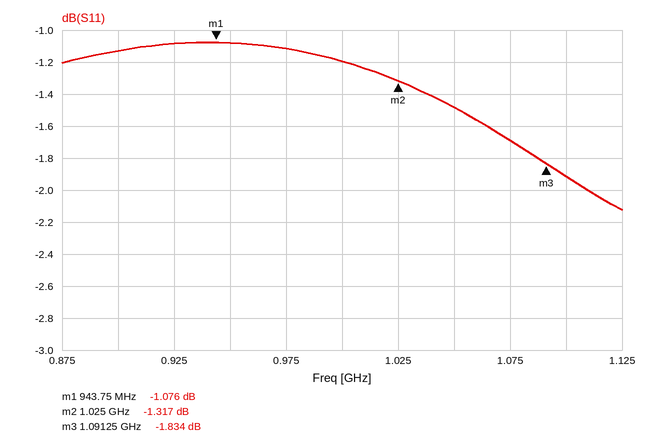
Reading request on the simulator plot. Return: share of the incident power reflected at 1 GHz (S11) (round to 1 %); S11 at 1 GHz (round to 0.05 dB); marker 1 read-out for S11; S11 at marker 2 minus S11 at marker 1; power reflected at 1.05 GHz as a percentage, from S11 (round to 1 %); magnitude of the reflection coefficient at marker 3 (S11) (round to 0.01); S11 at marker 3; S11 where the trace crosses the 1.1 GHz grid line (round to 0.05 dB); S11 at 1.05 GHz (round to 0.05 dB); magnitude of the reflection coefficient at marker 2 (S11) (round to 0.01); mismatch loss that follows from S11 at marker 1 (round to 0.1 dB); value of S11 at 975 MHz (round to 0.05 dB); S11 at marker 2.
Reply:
76 %
-1.20 dB
-1.076 dB
-0.241 dB
71 %
0.81
-1.834 dB
-1.90 dB
-1.50 dB
0.86
6.6 dB
-1.10 dB
-1.317 dB
